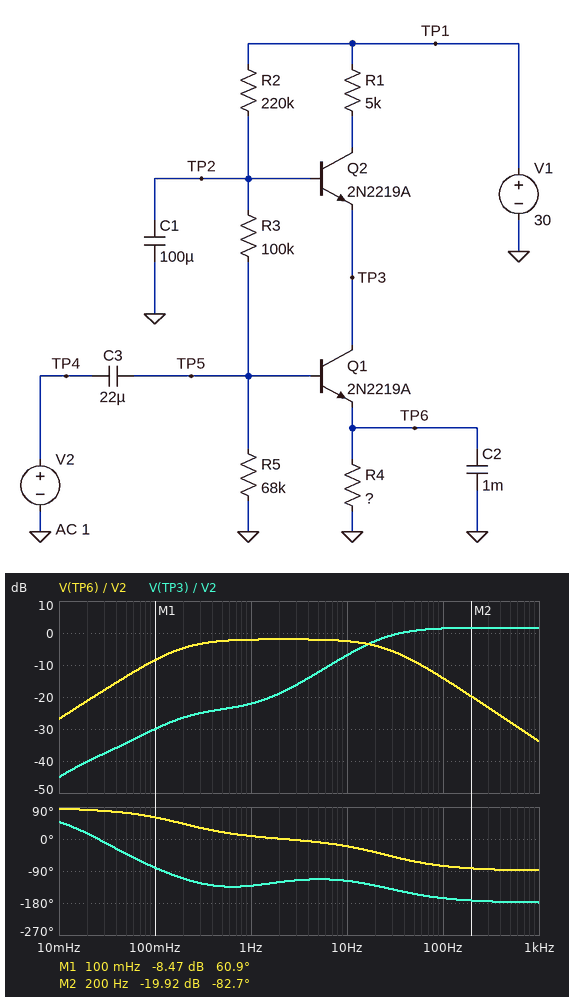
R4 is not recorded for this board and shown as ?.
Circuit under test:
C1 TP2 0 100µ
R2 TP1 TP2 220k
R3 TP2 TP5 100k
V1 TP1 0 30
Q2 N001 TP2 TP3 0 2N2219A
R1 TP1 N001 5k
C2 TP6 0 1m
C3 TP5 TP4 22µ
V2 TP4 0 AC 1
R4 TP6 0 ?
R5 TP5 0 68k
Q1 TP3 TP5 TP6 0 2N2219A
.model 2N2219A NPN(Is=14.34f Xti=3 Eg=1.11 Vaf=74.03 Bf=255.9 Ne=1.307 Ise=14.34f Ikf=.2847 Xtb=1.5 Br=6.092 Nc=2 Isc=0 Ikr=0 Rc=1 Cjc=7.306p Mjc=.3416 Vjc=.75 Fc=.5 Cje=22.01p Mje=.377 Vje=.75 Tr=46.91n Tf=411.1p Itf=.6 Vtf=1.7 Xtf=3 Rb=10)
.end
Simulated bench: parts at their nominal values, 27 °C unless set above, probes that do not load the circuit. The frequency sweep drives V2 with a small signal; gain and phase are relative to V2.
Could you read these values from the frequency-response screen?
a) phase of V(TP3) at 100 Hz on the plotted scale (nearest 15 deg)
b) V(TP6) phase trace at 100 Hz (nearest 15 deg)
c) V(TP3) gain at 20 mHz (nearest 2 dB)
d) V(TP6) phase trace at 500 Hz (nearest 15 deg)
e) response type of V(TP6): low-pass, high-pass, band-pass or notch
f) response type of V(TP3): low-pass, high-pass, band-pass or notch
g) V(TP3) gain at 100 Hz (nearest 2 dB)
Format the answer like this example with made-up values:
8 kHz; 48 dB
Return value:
-165 deg; -75 deg; -40 dB; -90 deg; band-pass; high-pass; 2 dB
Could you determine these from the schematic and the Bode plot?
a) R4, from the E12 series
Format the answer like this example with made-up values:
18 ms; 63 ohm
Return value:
820 Ω
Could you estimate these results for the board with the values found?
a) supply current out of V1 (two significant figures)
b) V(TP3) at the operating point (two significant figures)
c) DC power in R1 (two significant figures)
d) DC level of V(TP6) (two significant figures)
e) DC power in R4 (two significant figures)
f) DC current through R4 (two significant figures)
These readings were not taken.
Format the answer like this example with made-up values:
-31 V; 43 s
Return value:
3.4 mA; 9.7 V; 55 mW; 2.8 V; 9.3 mW; 3.4 mA
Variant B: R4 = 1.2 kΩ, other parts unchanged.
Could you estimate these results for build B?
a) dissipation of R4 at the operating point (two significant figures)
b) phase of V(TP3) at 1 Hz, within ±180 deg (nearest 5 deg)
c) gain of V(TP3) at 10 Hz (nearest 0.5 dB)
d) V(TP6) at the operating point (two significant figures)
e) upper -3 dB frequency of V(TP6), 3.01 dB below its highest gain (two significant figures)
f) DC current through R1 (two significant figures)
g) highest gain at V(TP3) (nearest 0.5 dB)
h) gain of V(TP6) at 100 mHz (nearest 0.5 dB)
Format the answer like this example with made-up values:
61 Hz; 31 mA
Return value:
8.3 mW; -125 deg; -5.5 dB; 3.2 V; 20 Hz; 2.6 mA; 1.5 dB; -8.0 dB
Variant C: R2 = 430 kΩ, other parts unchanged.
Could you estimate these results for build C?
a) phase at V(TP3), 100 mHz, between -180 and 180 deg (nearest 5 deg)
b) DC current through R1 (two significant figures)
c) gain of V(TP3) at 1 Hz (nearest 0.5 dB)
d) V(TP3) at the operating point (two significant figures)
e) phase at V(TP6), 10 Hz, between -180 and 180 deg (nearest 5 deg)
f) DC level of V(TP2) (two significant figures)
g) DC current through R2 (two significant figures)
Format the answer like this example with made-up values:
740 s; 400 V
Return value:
-70 deg; 1.9 mA; -20.5 dB; 6.0 V; -35 deg; 6.6 V; 54 µA
